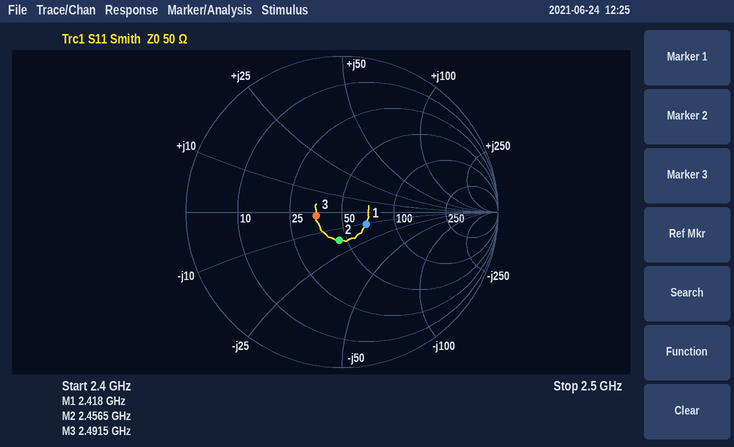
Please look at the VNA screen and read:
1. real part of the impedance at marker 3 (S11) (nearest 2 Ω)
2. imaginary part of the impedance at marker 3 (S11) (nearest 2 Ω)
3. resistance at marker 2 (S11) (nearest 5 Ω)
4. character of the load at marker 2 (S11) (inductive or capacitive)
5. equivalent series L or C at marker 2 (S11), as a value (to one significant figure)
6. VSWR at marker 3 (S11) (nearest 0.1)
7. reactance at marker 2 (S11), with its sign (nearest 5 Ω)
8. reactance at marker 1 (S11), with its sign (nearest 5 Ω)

36 Ω
-2 Ω
45 Ω
capacitive
4 pF
1.4
-15 Ω
-10 Ω
